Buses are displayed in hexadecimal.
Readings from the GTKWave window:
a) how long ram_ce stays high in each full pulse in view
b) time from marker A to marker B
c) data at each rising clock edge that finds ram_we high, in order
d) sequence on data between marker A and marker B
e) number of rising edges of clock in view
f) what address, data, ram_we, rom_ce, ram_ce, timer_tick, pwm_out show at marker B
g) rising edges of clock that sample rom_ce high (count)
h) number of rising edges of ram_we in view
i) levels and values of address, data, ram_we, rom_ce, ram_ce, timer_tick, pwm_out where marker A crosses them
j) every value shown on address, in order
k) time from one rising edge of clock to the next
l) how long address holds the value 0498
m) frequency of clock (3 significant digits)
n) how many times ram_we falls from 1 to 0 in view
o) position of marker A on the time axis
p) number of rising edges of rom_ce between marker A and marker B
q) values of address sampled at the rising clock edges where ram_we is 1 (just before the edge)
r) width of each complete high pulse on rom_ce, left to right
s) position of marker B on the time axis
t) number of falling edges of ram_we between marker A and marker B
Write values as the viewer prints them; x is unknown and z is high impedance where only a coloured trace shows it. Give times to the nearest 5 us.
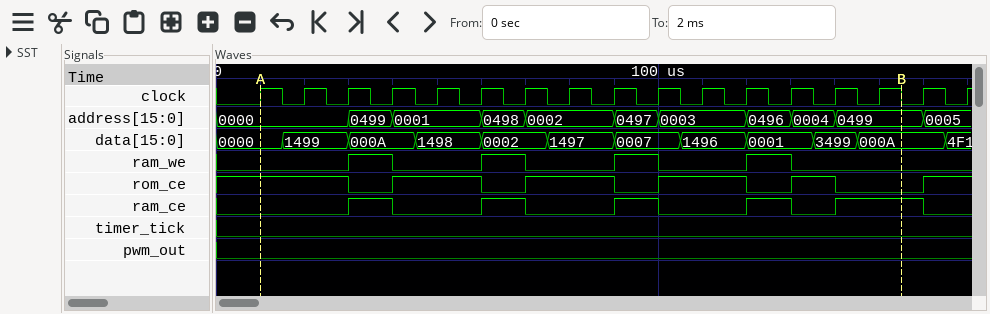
10 us, 10 us, 10 us, 10 us, 20 us
145 us
000A, 0002, 0007, 0001
0000, 1499, 000A, 1498, 0002, 1497, 0007, 1496, 0001, 3499, 000A
17
address=0499, data=000A, ram_we=0, rom_ce=0, ram_ce=1, timer_tick=0, pwm_out=0
11
4
address=0000, data=0000, ram_we=0, rom_ce=1, ram_ce=0, timer_tick=0, pwm_out=0
0000, 0499, 0001, 0498, 0002, 0497, 0003, 0496, 0004, 0499, 0005
10 us
10 us
100 kHz
4
10 us
4
0499, 0498, 0497, 0496
20 us, 20 us, 20 us, 10 us
155 us
4
